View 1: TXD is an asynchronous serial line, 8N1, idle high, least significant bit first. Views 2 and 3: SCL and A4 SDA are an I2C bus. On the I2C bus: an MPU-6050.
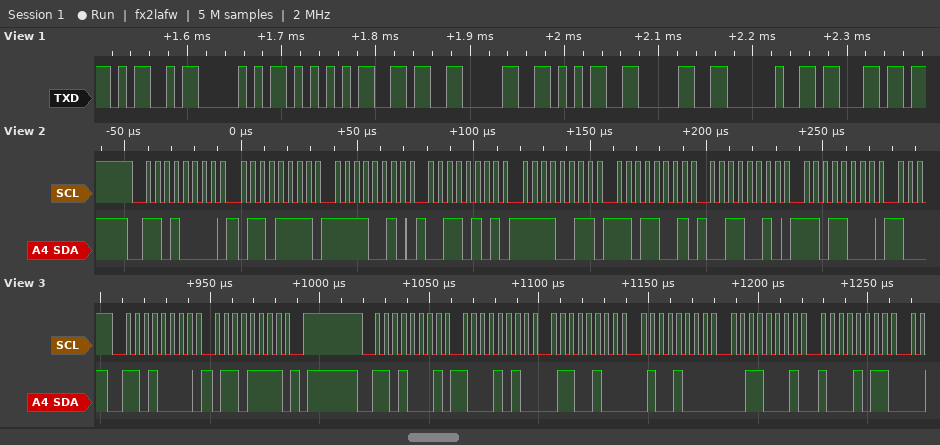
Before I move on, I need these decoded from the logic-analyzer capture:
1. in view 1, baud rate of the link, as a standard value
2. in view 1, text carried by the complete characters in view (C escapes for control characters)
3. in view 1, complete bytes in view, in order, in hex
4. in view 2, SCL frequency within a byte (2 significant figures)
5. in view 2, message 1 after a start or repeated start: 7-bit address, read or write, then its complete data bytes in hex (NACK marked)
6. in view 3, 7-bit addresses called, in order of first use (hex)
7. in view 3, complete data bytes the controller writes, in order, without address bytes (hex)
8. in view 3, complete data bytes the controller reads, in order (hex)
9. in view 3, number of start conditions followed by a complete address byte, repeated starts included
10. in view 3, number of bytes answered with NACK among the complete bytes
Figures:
115200 baud
"MPU6050 c"
4D 50 55 36 30 35 30 20 63
250 kHz
0x68 write: 6F F2 35 F3 D9 32 D8
0x68
6F
8A 64 48 31 8B
2
0
